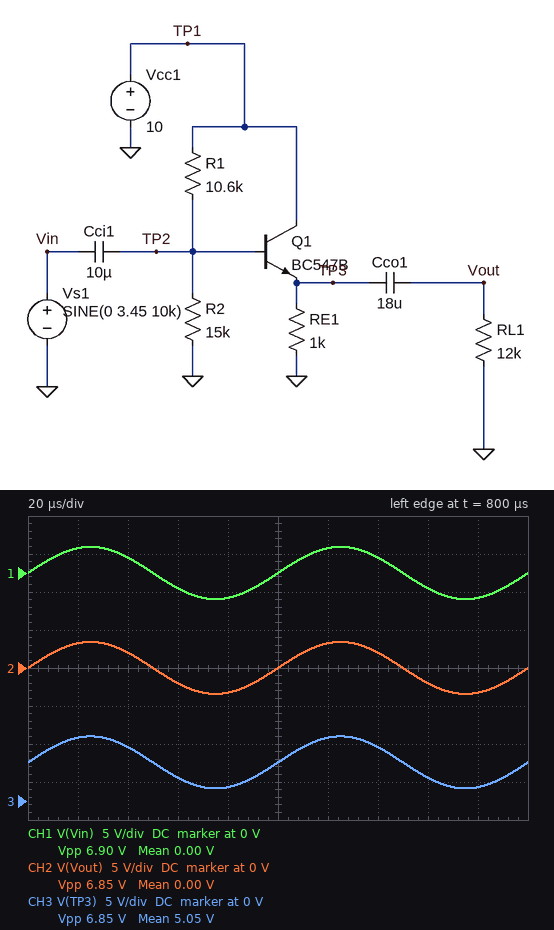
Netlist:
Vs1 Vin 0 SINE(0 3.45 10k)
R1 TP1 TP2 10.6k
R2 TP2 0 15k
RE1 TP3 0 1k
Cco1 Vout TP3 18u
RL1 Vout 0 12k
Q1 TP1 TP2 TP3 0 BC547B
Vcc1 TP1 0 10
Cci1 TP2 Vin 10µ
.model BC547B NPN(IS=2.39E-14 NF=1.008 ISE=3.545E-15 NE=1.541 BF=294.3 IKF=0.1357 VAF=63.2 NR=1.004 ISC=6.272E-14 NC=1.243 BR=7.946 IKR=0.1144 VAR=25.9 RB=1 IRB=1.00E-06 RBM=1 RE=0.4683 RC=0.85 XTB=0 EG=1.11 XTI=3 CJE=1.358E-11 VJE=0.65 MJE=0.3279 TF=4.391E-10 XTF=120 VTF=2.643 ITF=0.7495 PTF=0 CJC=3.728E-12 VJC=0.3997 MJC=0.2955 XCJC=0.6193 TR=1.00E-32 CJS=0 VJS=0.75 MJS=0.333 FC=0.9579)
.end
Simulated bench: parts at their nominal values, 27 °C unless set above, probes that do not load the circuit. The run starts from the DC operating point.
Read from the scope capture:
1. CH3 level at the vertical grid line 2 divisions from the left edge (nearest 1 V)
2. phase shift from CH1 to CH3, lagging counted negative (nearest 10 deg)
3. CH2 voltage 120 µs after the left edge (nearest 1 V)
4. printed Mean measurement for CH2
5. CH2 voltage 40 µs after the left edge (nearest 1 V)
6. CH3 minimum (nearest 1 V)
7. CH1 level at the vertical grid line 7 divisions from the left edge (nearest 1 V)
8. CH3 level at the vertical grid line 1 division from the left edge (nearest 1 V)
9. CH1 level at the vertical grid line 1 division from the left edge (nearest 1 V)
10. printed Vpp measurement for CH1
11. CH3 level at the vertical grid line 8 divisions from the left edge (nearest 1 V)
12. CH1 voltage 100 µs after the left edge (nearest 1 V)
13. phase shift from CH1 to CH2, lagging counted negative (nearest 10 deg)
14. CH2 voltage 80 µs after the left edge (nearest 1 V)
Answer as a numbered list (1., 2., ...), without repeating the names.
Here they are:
1. 7 V
2. 0 deg
3. 3 V
4. 0.00 V
5. 2 V
6. 2 V
7. 2 V
8. 8 V
9. 3 V
10. 6.90 V
11. 3 V
12. 0 V
13. 0 deg
14. -3 V
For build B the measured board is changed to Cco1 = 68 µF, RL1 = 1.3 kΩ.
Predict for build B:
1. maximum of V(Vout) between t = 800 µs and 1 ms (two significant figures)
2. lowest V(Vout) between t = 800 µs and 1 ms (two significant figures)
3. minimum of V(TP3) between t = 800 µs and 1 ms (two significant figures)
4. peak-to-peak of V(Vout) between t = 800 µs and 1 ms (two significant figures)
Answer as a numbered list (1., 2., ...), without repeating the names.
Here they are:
1. 3.4 V
2. -2.9 V
3. 2.2 V
4. 6.3 V
